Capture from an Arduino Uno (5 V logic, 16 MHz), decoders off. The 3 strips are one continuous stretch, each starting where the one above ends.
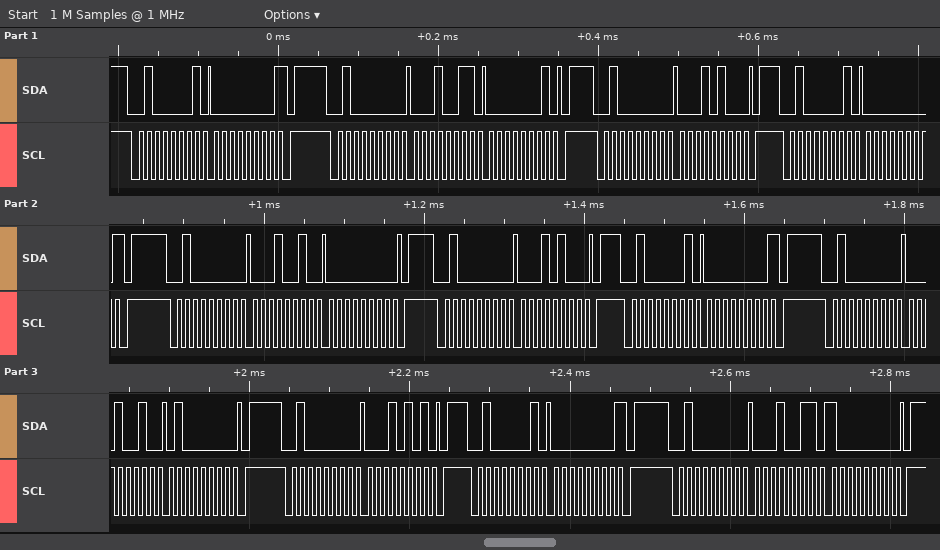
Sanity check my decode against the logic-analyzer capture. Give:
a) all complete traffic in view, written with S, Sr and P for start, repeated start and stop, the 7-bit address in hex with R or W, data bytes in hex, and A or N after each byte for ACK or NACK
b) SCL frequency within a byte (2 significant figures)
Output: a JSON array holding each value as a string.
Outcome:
["S 20R A 00 N P S 20W A 13 A 01 A P S 20W A 14 A P S 20R A 00 N P S 20W A 12 A 00 A P S 20W A 14 A P S 20R A 00 N P S 20W A 12 A 40 A P S 20W A 15 A P S 20R A 00 N P S 20W A 13 A 80 A P", "100 kHz"]
